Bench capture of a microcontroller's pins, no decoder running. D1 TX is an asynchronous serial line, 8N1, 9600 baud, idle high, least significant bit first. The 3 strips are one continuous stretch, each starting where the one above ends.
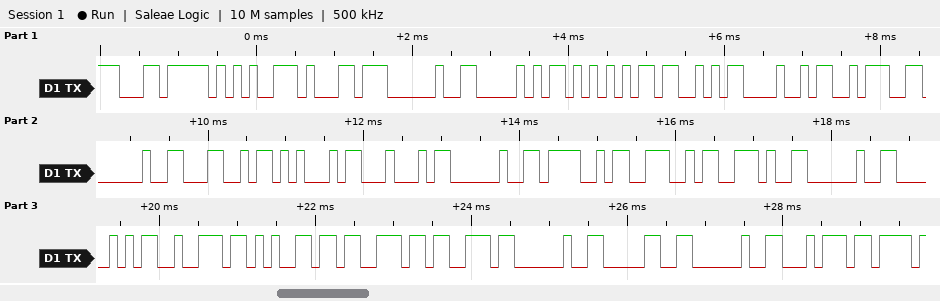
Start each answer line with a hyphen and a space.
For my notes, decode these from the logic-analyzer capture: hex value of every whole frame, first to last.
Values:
- EC 95 B1 20 50 55 53 48 3A 20 4C 45 44 20 4F 4E 2E 20 50 72 65 73 73 20 30 20 74
